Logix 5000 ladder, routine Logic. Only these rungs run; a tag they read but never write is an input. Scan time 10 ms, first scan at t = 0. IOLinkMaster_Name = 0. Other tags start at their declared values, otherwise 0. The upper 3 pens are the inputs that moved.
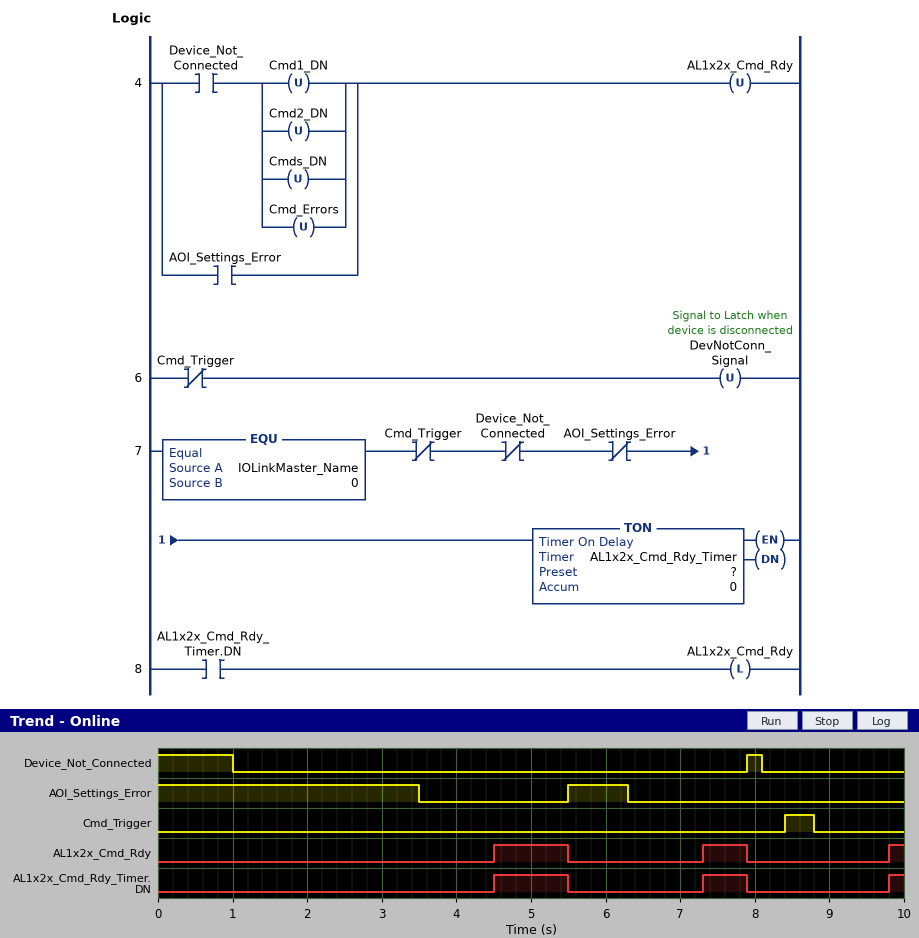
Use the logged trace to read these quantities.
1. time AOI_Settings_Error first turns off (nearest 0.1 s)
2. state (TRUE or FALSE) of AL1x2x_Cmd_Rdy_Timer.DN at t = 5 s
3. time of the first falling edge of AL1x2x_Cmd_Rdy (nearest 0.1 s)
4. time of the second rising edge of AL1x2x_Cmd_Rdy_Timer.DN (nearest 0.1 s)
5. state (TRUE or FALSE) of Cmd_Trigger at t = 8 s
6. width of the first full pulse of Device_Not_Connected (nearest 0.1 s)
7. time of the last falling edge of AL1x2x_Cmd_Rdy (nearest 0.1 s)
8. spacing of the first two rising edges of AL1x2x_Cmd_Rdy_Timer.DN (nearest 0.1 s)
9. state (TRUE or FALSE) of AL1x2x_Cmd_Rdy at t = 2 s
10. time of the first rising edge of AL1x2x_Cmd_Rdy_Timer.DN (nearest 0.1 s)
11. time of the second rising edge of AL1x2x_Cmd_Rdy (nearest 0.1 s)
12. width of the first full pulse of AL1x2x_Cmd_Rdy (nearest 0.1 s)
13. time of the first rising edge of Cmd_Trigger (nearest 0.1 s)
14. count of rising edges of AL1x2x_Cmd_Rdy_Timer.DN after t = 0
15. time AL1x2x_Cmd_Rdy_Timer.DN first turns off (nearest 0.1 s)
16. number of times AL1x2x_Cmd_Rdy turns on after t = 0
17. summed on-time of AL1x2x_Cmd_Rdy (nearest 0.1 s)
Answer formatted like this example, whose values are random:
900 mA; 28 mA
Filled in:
3.5 s; TRUE; 5.5 s; 7.3 s; FALSE; 0.2 s; 7.9 s; 2.8 s; FALSE; 4.5 s; 7.3 s; 1.0 s; 8.4 s; 3; 5.5 s; 3; 1.8 s
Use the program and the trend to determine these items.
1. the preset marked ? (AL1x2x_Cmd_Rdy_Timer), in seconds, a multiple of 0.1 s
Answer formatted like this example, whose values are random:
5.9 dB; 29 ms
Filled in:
1.0 s
